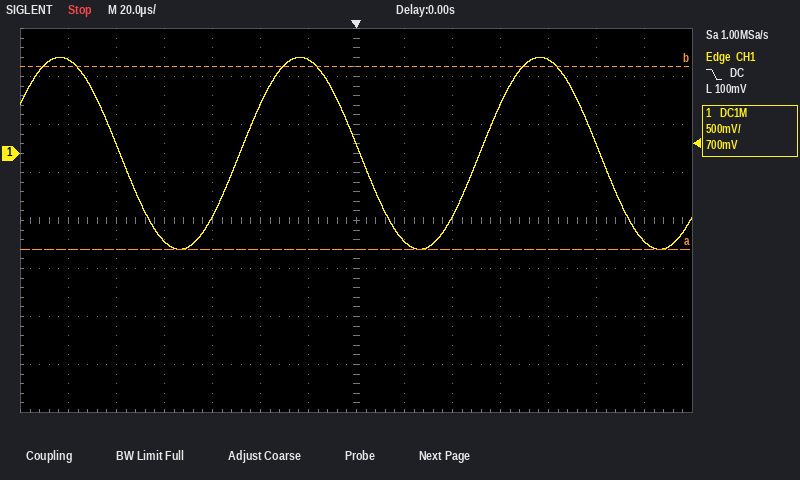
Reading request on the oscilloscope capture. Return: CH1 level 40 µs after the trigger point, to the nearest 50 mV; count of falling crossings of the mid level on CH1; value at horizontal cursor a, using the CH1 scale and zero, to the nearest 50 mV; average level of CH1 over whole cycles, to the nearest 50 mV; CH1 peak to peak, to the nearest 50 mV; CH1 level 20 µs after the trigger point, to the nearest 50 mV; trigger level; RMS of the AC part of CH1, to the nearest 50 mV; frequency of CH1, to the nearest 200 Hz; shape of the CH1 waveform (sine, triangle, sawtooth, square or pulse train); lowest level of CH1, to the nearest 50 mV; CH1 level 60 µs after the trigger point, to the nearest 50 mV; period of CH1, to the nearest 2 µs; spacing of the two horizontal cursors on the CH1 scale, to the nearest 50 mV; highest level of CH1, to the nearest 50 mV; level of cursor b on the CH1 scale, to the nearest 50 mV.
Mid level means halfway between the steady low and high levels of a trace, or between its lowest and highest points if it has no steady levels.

-650 mV
3
-1.00 V
0 mV
2.00 V
-900 mV
100 mV
700 mV
10.0 kHz
sine
-1.00 V
500 mV
100 µs
1.90 V
1.00 V
900 mV
